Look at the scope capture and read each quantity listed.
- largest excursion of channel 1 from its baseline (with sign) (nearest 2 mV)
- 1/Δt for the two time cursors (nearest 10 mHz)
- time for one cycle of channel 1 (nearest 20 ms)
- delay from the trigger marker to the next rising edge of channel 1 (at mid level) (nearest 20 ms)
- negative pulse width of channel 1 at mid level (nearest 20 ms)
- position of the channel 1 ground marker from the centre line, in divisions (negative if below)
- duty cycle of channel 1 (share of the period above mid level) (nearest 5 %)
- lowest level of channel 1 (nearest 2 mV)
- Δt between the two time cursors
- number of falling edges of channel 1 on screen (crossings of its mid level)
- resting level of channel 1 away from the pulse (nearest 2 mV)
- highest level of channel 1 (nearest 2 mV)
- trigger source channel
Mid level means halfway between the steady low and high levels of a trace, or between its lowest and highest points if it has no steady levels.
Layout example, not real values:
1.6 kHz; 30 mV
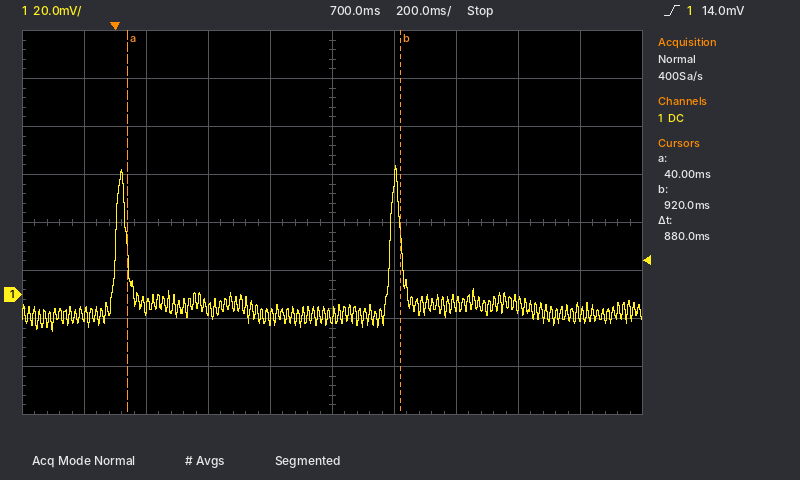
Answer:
+60 mV; 1.14 Hz; 880 ms; 880 ms; 840 ms; -1.5 div; 5 %; -16 mV; 880 ms; 2; -6 mV; 54 mV; channel 1
